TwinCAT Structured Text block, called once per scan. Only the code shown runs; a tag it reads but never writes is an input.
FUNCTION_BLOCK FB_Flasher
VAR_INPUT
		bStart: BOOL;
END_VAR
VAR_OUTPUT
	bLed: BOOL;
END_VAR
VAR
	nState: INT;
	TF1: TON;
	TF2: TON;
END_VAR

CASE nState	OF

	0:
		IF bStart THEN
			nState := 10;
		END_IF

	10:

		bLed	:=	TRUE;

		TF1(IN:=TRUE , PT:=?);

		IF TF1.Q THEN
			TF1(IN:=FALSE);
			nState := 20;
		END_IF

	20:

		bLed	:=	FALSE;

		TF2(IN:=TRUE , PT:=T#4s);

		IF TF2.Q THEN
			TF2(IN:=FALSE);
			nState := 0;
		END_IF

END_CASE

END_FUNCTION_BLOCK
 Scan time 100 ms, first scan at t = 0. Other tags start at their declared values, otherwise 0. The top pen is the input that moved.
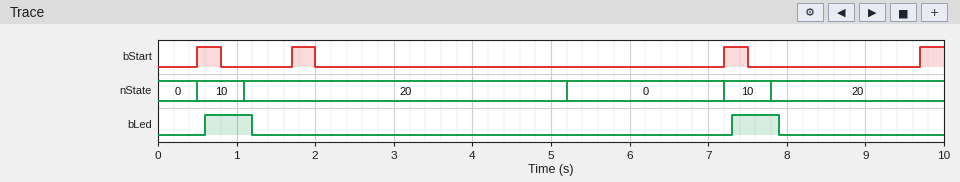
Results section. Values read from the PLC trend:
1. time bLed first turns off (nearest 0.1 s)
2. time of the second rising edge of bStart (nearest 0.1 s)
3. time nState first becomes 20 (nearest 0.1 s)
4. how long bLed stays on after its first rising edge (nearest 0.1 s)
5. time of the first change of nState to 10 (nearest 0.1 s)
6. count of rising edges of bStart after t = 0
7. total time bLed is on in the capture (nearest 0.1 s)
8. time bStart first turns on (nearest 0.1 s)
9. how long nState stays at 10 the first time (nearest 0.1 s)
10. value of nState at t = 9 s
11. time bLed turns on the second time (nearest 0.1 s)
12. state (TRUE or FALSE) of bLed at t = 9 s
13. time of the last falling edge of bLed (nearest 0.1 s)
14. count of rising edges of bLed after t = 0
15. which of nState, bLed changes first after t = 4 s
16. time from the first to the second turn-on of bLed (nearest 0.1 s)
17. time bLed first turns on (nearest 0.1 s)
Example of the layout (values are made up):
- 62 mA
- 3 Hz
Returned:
- 1.2 s
- 1.7 s
- 1.1 s
- 0.6 s
- 0.5 s
- 4
- 1.2 s
- 0.5 s
- 0.6 s
- 20
- 7.3 s
- FALSE
- 7.9 s
- 2
- nState
- 6.7 s
- 0.6 s
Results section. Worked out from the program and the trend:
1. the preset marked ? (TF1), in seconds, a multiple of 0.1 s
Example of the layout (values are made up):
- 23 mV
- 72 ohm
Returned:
- 0.5 s
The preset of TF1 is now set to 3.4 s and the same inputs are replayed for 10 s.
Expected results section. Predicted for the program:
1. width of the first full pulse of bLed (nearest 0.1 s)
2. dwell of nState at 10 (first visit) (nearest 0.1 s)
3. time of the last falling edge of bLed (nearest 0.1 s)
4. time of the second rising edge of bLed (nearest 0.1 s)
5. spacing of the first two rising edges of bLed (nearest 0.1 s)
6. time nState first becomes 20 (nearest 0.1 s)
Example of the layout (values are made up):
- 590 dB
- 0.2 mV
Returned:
- 3.5 s
- 3.5 s
- 4.1 s
- 9.8 s
- 9.2 s
- 4.0 s
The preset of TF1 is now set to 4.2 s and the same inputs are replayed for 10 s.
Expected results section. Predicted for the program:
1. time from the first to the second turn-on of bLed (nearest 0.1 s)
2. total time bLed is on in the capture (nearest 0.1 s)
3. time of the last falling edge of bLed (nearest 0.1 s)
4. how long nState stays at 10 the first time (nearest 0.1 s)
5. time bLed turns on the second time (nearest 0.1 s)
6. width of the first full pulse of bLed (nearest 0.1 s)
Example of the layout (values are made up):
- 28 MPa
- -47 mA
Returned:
- 9.2 s
- 4.5 s
- 4.9 s
- 4.3 s
- 9.8 s
- 4.3 s
